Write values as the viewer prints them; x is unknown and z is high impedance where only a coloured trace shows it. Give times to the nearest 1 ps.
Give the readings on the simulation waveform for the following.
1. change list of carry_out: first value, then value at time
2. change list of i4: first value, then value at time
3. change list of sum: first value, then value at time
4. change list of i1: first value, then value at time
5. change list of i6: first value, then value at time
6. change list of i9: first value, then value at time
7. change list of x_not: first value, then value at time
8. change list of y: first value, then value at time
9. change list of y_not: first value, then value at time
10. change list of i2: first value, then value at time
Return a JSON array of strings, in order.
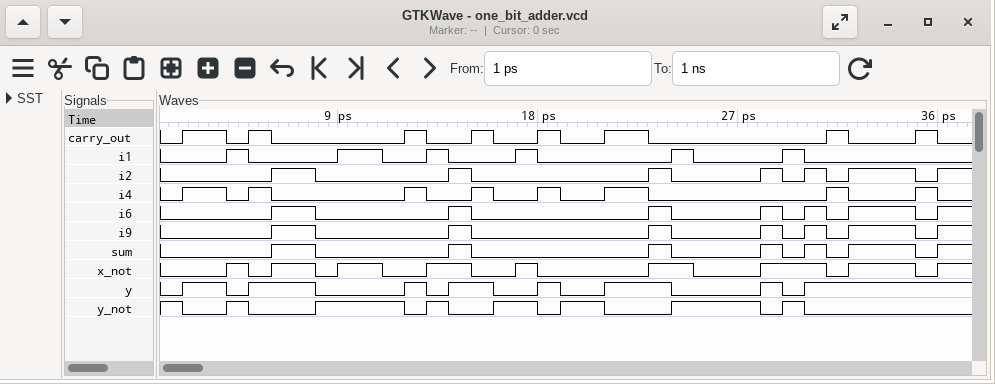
["0, 1 at 2 ps, 0 at 4 ps, 1 at 5 ps, 0 at 6 ps, 1 at 12 ps, 0 at 13 ps, 1 at 15 ps, 0 at 16 ps, 1 at 18 ps, 0 at 19 ps, 1 at 21 ps, 0 at 23 ps, 1 at 31 ps, 0 at 32 ps, 1 at 35 ps, 0 at 36 ps", "0, 1 at 2 ps, 0 at 4 ps, 1 at 5 ps, 0 at 6 ps, 1 at 12 ps, 0 at 13 ps, 1 at 15 ps, 0 at 16 ps, 1 at 18 ps, 0 at 19 ps, 1 at 21 ps, 0 at 23 ps, 1 at 31 ps, 0 at 32 ps, 1 at 35 ps, 0 at 36 ps", "0, 1 at 6 ps, 0 at 8 ps, 1 at 14 ps, 0 at 15 ps, 1 at 23 ps, 0 at 24 ps, 1 at 28 ps, 0 at 29 ps, 1 at 30 ps, 0 at 31 ps, 1 at 32 ps, 0 at 35 ps, 1 at 36 ps", "0, 1 at 4 ps, 0 at 5 ps, 1 at 9 ps, 0 at 11 ps, 1 at 13 ps, 0 at 14 ps, 1 at 17 ps, 0 at 18 ps, 1 at 24 ps, 0 at 25 ps, 1 at 29 ps, 0 at 30 ps", "0, 1 at 6 ps, 0 at 8 ps, 1 at 14 ps, 0 at 15 ps, 1 at 23 ps, 0 at 24 ps, 1 at 28 ps, 0 at 29 ps, 1 at 30 ps, 0 at 31 ps, 1 at 32 ps, 0 at 35 ps, 1 at 36 ps", "0, 1 at 6 ps, 0 at 8 ps, 1 at 14 ps, 0 at 15 ps, 1 at 23 ps, 0 at 24 ps, 1 at 28 ps, 0 at 29 ps, 1 at 30 ps, 0 at 31 ps, 1 at 32 ps, 0 at 35 ps, 1 at 36 ps", "0, 1 at 4 ps, 0 at 5 ps, 1 at 6 ps, 0 at 8 ps, 1 at 9 ps, 0 at 11 ps, 1 at 13 ps, 0 at 15 ps, 1 at 17 ps, 0 at 18 ps, 1 at 23 ps, 0 at 25 ps, 1 at 28 ps, 0 at 31 ps, 1 at 32 ps, 0 at 35 ps, 1 at 36 ps", "0, 1 at 2 ps, 0 at 4 ps, 1 at 5 ps, 0 at 8 ps, 1 at 12 ps, 0 at 13 ps, 1 at 14 ps, 0 at 16 ps, 1 at 18 ps, 0 at 19 ps, 1 at 21 ps, 0 at 24 ps, 1 at 28 ps, 0 at 29 ps, 1 at 30 ps", "1, 0 at 2 ps, 1 at 4 ps, 0 at 5 ps, 1 at 8 ps, 0 at 12 ps, 1 at 13 ps, 0 at 14 ps, 1 at 16 ps, 0 at 18 ps, 1 at 19 ps, 0 at 21 ps, 1 at 24 ps, 0 at 28 ps, 1 at 29 ps, 0 at 30 ps", "0, 1 at 6 ps, 0 at 8 ps, 1 at 14 ps, 0 at 15 ps, 1 at 23 ps, 0 at 24 ps, 1 at 28 ps, 0 at 29 ps, 1 at 30 ps, 0 at 31 ps, 1 at 32 ps, 0 at 35 ps, 1 at 36 ps"]
